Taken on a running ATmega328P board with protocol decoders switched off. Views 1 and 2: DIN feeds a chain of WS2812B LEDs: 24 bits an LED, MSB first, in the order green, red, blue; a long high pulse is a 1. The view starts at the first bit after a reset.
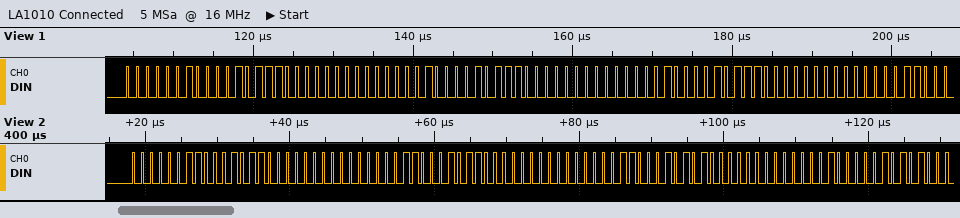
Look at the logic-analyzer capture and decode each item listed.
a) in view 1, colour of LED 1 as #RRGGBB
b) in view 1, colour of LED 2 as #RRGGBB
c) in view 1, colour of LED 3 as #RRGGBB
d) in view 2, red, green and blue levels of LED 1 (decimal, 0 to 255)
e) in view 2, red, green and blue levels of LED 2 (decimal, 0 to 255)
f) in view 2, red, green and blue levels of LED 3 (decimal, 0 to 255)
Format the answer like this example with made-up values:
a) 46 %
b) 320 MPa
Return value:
a) #170200
b) #170200
c) #170200
d) 22, 3, 0
e) 22, 3, 0
f) 21, 3, 0
